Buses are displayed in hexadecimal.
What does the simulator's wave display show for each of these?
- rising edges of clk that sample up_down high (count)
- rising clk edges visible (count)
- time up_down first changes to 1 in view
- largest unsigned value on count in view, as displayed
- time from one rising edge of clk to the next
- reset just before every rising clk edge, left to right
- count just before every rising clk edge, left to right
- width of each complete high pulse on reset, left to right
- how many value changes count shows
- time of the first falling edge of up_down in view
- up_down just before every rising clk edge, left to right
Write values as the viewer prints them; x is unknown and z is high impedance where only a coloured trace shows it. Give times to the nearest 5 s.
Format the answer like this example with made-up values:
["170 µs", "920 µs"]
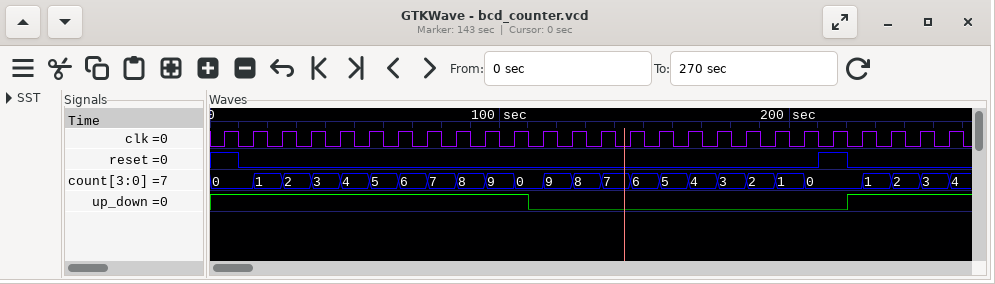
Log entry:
["15", "26", "220 s", "9", "10 s", "1 0 0 0 0 0 0 0 0 0 0 0 0 0 0 0 0 0 0 0 0 1 0 0 0 0", "0, 0, 1, 2, 3, 4, 5, 6, 7, 8, 9, 0, 9, 8, 7, 6, 5, 4, 3, 2, 1, 0, 0, 1, 2, 3", "10 s", "24", "110 s", "1 1 1 1 1 1 1 1 1 1 1 0 0 0 0 0 0 0 0 0 0 0 1 1 1 1"]
